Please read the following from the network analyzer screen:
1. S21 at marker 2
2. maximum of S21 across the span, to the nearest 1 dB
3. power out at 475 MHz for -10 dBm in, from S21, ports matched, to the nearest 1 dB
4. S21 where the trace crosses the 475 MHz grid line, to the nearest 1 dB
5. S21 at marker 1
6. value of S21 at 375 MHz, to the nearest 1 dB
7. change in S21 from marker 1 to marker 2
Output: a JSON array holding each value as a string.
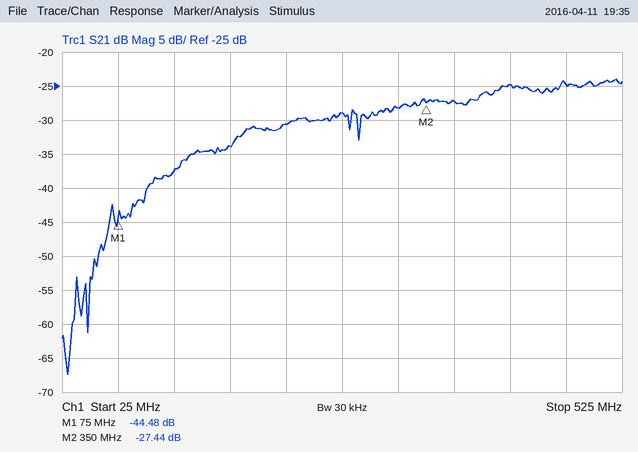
["-27.44 dB", "-24 dB", "-35 dBm", "-25 dB", "-44.48 dB", "-27 dB", "17.04 dB"]
